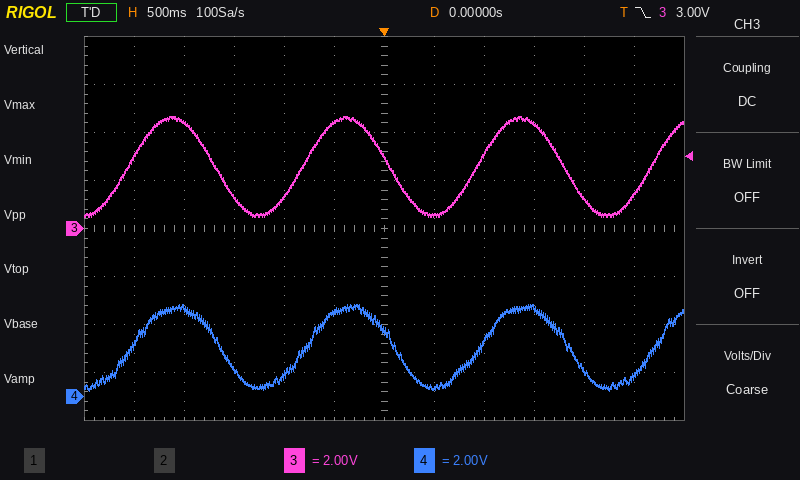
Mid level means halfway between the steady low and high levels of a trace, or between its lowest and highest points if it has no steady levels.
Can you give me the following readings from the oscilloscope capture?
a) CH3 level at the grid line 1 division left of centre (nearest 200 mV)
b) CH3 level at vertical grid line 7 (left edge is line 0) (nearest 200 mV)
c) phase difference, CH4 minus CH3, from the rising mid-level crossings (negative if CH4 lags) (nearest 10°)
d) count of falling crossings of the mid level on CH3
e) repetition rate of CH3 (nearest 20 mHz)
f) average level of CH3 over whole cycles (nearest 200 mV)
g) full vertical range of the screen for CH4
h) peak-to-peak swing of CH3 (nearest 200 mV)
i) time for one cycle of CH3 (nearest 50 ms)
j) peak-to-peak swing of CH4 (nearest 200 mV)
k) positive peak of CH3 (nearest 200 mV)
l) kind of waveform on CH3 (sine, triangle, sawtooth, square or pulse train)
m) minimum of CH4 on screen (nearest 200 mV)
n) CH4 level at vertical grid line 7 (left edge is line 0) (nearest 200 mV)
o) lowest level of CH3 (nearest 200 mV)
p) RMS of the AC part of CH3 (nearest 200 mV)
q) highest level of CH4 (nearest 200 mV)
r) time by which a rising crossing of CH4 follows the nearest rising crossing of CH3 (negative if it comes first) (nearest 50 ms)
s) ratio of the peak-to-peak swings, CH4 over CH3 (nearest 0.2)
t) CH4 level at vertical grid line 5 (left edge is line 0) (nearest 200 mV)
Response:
4.4 V
600 mV
-10°
3
580 mHz
2.6 V
16 V
4.2 V
1.75 s
3.6 V
4.6 V
sine
200 mV
400 mV
400 mV
1.4 V
3.8 V
+50 ms
0.8
3.6 V
